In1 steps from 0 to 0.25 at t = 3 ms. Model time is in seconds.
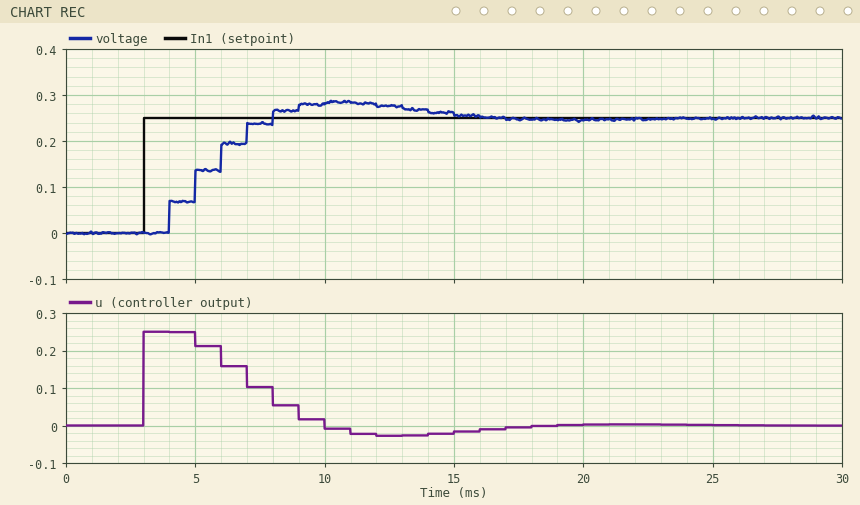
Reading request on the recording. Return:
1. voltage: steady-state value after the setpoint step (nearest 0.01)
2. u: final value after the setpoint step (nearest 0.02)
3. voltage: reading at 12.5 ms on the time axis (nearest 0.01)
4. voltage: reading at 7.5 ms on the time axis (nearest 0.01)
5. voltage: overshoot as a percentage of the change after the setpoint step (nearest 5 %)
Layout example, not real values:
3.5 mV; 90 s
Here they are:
0.25; 0.00; 0.28; 0.24; 15 %
